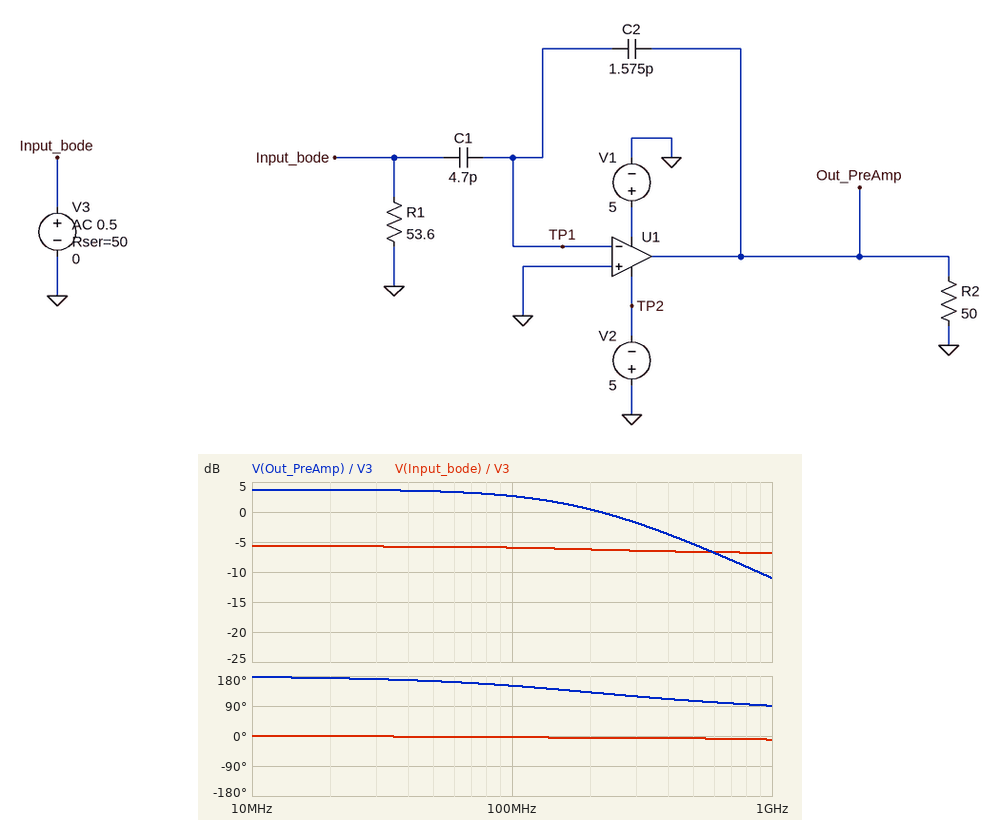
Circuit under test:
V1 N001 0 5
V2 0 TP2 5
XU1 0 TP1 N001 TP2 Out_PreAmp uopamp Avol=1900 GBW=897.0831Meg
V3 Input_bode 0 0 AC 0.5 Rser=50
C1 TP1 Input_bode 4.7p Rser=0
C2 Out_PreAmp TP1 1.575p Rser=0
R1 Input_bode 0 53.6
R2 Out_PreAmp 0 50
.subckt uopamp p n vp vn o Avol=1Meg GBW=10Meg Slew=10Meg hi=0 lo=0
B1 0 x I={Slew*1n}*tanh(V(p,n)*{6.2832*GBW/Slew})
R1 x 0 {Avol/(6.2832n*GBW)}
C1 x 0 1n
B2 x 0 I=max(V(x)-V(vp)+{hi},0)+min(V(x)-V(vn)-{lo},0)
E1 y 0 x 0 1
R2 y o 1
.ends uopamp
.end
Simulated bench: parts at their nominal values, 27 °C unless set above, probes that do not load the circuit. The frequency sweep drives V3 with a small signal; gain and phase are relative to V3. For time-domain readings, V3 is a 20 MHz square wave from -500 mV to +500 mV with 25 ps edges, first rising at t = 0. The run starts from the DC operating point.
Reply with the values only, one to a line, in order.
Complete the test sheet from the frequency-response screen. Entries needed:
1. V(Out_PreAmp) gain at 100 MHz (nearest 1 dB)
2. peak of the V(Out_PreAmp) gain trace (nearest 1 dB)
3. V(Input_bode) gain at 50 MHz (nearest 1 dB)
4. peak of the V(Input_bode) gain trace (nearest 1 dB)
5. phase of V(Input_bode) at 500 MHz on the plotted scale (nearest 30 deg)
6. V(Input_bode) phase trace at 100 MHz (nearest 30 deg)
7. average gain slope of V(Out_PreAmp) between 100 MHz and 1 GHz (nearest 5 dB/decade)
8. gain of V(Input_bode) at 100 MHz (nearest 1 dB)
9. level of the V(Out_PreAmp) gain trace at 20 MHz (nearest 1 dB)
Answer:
3 dB
4 dB
-6 dB
-6 dB
0 deg
0 deg
-15 dB/decade
-6 dB
4 dB
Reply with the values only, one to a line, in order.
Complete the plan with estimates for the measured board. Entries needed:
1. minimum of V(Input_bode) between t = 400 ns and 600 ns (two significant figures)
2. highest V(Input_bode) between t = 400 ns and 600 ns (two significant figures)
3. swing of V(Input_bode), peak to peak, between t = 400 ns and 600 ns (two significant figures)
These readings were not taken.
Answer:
-260 mV
260 mV
520 mV
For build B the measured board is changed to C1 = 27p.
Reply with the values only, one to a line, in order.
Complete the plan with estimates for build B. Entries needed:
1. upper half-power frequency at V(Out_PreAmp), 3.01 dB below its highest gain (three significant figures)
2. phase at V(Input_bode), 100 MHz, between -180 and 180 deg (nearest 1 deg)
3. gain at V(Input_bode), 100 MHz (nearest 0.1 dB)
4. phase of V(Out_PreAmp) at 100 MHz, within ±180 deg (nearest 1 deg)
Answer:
40.7 MHz
-5 deg
-7.1 dB
111 deg
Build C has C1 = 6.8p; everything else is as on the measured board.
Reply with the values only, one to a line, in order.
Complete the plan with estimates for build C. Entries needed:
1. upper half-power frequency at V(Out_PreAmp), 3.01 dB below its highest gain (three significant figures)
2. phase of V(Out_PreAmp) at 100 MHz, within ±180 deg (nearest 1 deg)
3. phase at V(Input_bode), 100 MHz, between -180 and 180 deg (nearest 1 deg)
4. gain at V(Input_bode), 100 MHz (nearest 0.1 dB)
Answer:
144 MHz
144 deg
-5 deg
-6.1 dB
